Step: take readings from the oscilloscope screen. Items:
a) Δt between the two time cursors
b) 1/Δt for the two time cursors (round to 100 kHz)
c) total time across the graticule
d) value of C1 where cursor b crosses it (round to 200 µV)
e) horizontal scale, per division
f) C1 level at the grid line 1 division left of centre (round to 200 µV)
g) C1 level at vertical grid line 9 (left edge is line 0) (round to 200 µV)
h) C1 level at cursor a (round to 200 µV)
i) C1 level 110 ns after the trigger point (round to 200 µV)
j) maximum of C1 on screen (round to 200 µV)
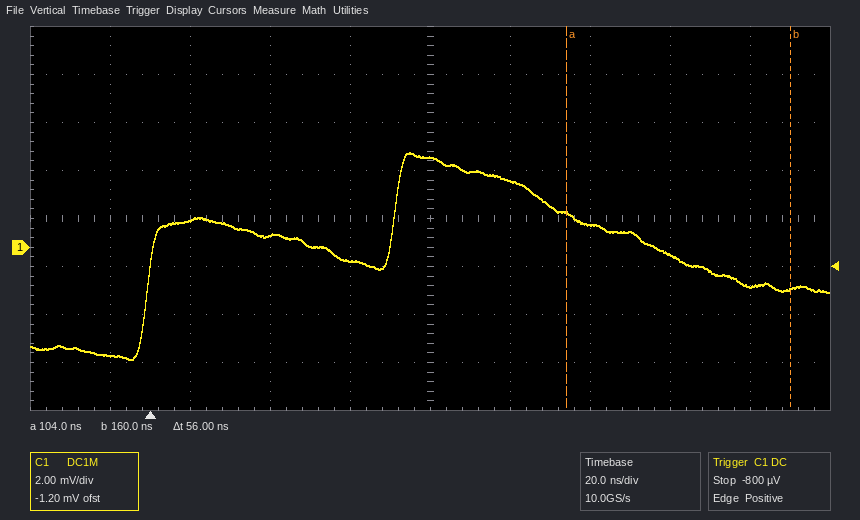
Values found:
56 ns
17.9 MHz
200 ns
-1.8 mV
20 ns
-600 µV
-1.6 mV
1.4 mV
1.0 mV
4.0 mV
